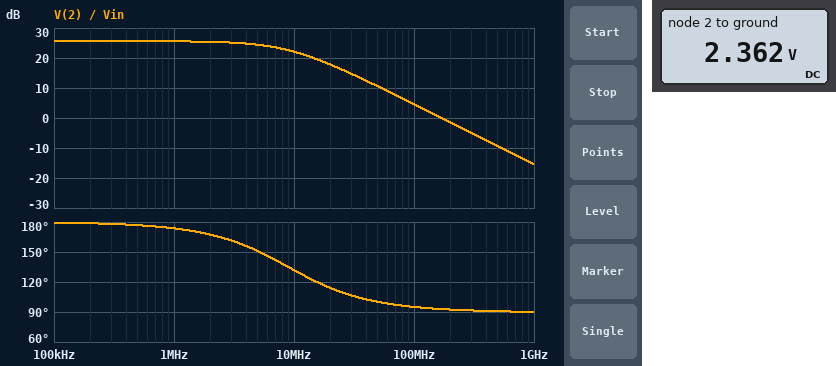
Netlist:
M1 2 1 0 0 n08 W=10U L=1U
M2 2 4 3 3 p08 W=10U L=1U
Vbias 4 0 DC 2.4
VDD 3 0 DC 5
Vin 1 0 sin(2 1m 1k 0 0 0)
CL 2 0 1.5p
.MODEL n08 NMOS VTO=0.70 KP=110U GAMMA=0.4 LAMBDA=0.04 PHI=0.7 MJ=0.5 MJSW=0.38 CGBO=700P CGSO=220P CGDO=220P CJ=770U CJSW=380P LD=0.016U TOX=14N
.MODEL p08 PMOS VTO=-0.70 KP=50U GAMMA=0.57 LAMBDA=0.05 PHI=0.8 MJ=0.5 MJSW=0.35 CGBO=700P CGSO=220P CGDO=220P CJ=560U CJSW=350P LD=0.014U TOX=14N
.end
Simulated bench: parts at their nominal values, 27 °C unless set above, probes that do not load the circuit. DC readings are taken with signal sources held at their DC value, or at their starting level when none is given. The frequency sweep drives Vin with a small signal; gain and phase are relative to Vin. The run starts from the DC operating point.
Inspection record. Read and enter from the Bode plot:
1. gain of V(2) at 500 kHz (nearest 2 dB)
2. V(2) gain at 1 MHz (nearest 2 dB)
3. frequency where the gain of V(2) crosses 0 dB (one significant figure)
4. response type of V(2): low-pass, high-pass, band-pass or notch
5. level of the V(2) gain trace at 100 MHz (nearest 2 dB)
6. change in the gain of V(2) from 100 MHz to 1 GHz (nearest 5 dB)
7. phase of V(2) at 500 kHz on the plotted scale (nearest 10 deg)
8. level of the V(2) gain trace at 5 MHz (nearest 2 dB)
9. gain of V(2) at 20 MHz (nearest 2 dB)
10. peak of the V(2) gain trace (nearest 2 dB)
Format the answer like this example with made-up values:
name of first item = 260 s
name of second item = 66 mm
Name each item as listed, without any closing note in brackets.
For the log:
gain of V(2) at 500 kHz = 26 dB
V(2) gain at 1 MHz = 26 dB
frequency where the gain of V(2) crosses 0 dB = 200 MHz
response type of V(2): low-pass, high-pass, band-pass or notch = low-pass
level of the V(2) gain trace at 100 MHz = 4 dB
change in the gain of V(2) from 100 MHz to 1 GHz = -20 dB
phase of V(2) at 500 kHz on the plotted scale = 180 deg
level of the V(2) gain trace at 5 MHz = 24 dB
gain of V(2) at 20 MHz = 18 dB
peak of the V(2) gain trace = 26 dB
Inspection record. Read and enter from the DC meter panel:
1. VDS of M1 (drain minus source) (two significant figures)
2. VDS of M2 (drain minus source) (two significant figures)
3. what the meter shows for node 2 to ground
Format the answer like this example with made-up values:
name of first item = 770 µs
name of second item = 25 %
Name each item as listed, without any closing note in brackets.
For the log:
VDS of M1 (drain minus source) = 2.4 V
VDS of M2 (drain minus source) = -2.6 V
what the meter shows for node 2 to ground = 2.362 V
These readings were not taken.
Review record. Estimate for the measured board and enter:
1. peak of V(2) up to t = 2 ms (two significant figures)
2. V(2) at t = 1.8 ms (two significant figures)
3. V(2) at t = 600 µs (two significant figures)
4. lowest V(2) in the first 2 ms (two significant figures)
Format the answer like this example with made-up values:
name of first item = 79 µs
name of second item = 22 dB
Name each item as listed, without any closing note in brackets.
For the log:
peak of V(2) up to t = 2 ms = 2.4 V
V(2) at t = 1.8 ms = 2.4 V
V(2) at t = 600 µs = 2.4 V
lowest V(2) in the first 2 ms = 2.3 V
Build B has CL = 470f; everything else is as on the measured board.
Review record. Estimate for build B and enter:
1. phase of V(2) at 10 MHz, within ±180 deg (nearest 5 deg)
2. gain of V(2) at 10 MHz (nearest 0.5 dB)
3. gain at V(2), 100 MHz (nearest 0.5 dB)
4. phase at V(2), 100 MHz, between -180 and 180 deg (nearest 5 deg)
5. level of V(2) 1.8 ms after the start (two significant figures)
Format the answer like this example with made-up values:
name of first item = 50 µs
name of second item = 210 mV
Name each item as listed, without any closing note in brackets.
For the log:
phase of V(2) at 10 MHz, within ±180 deg = 160 deg
gain of V(2) at 10 MHz = 25.0 dB
gain at V(2), 100 MHz = 14.5 dB
phase at V(2), 100 MHz, between -180 and 180 deg = 105 deg
level of V(2) 1.8 ms after the start = 2.4 V
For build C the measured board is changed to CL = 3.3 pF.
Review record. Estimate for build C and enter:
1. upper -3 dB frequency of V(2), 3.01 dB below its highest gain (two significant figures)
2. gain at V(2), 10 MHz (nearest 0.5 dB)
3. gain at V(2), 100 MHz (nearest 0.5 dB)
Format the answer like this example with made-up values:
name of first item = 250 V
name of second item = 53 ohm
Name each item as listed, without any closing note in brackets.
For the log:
upper -3 dB frequency of V(2), 3.01 dB below its highest gain = 4.1 MHz
gain at V(2), 10 MHz = 17.0 dB
gain at V(2), 100 MHz = -2.0 dB
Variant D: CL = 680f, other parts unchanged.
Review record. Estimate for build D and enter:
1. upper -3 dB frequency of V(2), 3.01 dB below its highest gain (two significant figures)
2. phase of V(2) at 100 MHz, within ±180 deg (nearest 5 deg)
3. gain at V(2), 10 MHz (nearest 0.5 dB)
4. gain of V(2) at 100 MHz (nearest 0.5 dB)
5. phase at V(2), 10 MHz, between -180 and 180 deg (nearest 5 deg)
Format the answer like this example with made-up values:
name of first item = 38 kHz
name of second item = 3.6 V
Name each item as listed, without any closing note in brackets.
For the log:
upper -3 dB frequency of V(2), 3.01 dB below its highest gain = 20 MHz
phase of V(2) at 100 MHz, within ±180 deg = 100 deg
gain at V(2), 10 MHz = 24.5 dB
gain of V(2) at 100 MHz = 11.5 dB
phase at V(2), 10 MHz, between -180 and 180 deg = 155 deg
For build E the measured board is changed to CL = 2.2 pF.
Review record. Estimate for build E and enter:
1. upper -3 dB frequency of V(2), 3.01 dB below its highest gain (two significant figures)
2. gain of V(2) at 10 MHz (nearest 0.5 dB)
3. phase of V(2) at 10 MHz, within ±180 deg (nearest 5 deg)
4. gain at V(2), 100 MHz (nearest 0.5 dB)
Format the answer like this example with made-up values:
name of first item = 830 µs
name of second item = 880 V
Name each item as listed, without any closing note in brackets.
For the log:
upper -3 dB frequency of V(2), 3.01 dB below its highest gain = 6.1 MHz
gain of V(2) at 10 MHz = 20.0 dB
phase of V(2) at 10 MHz, within ±180 deg = 120 deg
gain at V(2), 100 MHz = 1.5 dB
